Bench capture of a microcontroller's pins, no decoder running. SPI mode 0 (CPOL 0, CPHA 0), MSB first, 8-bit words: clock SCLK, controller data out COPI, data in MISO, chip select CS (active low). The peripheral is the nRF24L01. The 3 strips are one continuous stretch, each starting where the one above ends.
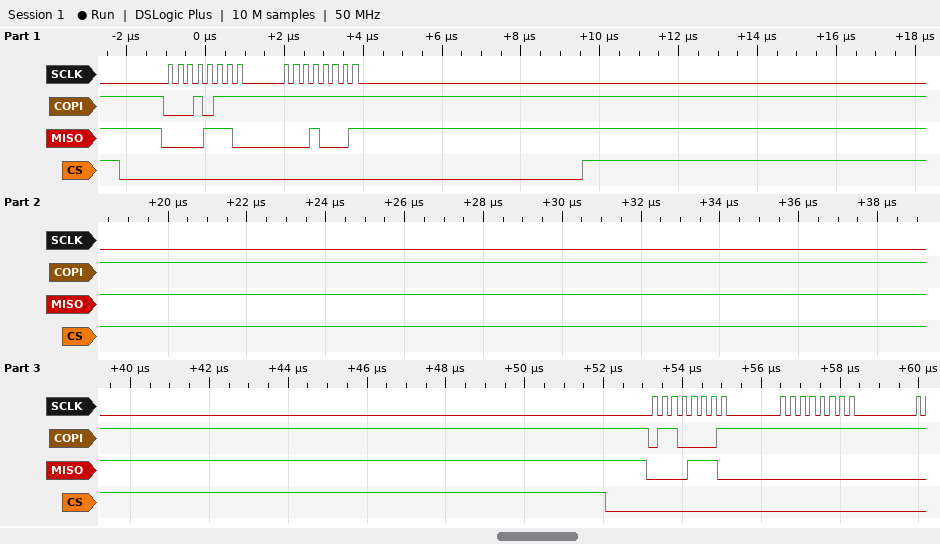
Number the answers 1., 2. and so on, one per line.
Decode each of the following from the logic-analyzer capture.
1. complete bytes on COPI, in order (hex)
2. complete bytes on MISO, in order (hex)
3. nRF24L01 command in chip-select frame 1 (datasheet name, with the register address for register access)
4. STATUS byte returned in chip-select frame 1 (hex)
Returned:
1. 17 FF 61 FF
2. 0E 11 0E 00
3. R_REGISTER 0x17
4. 0x0E
